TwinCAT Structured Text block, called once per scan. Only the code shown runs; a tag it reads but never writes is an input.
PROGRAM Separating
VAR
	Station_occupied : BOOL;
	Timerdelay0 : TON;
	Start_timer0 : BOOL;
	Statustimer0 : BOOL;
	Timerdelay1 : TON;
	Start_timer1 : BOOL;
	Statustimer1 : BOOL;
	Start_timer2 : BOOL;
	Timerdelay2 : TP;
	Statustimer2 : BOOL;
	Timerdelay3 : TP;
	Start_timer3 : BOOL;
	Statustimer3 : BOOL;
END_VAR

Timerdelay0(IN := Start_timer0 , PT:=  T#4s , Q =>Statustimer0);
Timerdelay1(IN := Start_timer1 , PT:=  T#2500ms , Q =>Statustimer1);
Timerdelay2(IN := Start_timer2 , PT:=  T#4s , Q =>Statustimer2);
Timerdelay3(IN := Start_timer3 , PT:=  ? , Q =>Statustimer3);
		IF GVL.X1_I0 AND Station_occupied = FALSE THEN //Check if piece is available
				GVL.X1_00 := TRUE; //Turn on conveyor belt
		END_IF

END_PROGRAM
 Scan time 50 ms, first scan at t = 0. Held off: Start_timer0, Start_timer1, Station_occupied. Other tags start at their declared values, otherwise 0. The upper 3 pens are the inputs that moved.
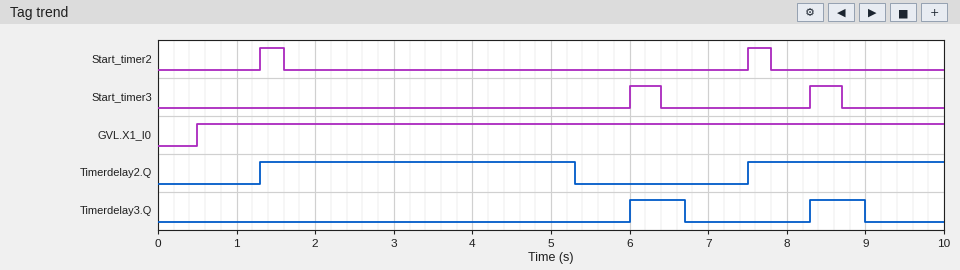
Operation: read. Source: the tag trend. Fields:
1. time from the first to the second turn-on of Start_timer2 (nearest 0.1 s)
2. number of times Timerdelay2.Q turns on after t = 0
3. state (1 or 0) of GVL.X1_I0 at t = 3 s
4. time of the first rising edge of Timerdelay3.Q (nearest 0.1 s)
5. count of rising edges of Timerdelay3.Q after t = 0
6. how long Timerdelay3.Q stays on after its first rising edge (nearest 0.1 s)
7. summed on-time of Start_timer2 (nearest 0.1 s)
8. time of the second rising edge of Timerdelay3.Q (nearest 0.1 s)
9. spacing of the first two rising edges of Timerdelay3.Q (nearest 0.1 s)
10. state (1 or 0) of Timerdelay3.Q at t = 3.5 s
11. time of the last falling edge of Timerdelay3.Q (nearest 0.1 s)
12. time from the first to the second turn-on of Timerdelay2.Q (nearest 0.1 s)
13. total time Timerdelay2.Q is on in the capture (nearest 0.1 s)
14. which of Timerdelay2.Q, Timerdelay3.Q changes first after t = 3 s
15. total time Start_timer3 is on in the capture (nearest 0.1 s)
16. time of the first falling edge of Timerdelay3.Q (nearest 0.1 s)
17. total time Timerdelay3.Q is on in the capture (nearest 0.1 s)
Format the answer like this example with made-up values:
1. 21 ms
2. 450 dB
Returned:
1. 6.2 s
2. 2
3. 1
4. 6.0 s
5. 2
6. 0.7 s
7. 0.6 s
8. 8.3 s
9. 2.3 s
10. 0
11. 9.0 s
12. 6.2 s
13. 6.5 s
14. Timerdelay2.Q
15. 0.8 s
16. 6.7 s
17. 1.4 s
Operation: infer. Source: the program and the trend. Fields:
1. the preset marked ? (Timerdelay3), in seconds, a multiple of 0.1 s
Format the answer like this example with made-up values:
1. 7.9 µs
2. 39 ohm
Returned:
1. 0.7 s
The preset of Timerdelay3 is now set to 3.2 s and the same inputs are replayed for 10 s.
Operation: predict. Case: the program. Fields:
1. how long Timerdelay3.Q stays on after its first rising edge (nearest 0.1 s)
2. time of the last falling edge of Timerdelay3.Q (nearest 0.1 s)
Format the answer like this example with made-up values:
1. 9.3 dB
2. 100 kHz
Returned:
1. 3.2 s
2. 9.2 s
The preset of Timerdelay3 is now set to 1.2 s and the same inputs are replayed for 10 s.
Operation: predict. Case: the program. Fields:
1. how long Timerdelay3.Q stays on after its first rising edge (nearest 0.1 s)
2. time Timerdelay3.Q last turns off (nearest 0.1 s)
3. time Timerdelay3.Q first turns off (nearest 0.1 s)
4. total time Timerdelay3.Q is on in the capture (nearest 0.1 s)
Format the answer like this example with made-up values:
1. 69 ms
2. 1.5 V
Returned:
1. 1.2 s
2. 9.5 s
3. 7.2 s
4. 2.4 s
